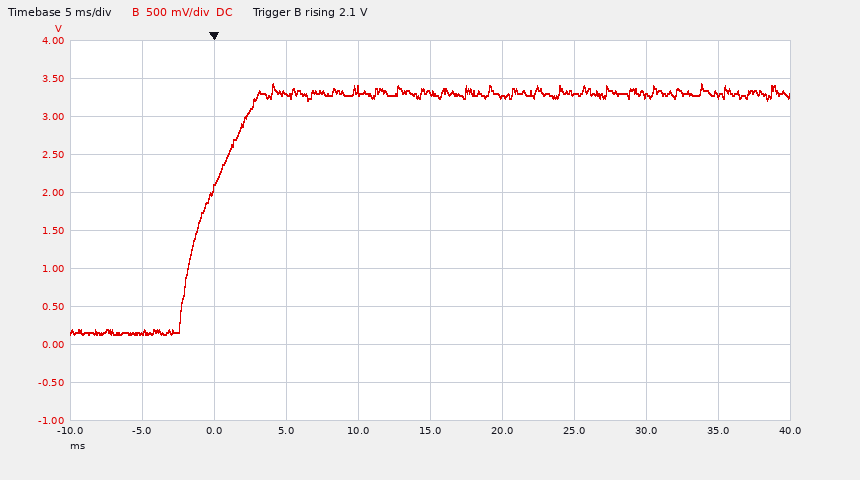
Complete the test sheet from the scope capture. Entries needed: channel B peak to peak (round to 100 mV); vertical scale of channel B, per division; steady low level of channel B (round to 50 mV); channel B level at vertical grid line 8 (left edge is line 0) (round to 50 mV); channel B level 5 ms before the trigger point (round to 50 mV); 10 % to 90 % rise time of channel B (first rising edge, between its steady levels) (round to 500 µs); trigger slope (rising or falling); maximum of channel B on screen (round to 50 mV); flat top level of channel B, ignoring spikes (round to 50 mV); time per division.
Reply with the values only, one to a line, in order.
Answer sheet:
3.30 V
500 mV
150 mV
3.30 V
150 mV
4.5 ms
rising
3.45 V
3.30 V
5 ms
